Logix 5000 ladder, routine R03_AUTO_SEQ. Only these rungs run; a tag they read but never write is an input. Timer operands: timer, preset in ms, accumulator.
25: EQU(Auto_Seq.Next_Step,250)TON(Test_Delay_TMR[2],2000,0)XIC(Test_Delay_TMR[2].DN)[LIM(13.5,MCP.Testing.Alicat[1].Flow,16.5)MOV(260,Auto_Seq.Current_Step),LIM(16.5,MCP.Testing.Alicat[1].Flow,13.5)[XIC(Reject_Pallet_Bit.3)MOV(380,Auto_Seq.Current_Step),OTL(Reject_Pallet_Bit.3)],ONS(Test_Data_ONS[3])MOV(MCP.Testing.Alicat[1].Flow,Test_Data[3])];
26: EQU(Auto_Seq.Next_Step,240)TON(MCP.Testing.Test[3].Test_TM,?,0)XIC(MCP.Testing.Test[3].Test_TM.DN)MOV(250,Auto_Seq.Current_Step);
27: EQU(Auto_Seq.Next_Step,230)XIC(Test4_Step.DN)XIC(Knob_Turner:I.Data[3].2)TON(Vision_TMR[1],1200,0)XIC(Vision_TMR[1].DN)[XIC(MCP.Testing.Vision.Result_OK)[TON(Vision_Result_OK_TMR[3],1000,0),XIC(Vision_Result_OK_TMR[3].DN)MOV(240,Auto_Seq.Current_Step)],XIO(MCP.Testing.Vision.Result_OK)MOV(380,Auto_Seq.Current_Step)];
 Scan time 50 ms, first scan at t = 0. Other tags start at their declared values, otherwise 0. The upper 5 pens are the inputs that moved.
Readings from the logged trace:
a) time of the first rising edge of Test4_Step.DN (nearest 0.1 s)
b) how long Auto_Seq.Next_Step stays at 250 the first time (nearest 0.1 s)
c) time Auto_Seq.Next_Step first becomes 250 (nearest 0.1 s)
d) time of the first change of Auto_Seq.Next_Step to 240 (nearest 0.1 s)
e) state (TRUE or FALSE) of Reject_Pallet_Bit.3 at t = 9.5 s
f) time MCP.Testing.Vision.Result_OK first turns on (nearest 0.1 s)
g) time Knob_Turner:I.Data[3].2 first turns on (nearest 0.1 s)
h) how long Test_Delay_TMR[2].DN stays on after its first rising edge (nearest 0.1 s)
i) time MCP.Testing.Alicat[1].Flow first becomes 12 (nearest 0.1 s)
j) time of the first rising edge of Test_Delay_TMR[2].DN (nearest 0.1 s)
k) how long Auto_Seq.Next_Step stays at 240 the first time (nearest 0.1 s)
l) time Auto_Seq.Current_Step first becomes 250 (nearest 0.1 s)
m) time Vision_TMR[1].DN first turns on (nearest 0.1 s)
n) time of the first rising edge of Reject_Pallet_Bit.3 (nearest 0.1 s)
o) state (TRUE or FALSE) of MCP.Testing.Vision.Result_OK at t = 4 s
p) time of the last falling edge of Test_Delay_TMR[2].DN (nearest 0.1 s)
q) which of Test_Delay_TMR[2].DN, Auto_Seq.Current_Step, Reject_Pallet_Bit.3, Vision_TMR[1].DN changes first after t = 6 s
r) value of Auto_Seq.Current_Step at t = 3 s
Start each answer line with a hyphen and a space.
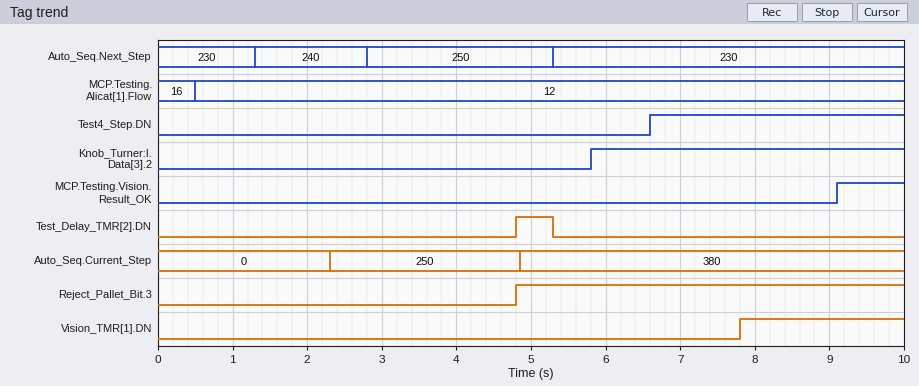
- 6.6 s
- 2.5 s
- 2.8 s
- 1.3 s
- TRUE
- 9.1 s
- 5.8 s
- 0.5 s
- 0.5 s
- 4.8 s
- 1.5 s
- 2.3 s
- 7.8 s
- 4.8 s
- FALSE
- 5.3 s
- Vision_TMR[1].DN
- 250
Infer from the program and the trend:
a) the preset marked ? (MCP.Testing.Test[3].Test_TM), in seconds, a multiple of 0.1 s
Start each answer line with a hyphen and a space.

- 1.0 s
